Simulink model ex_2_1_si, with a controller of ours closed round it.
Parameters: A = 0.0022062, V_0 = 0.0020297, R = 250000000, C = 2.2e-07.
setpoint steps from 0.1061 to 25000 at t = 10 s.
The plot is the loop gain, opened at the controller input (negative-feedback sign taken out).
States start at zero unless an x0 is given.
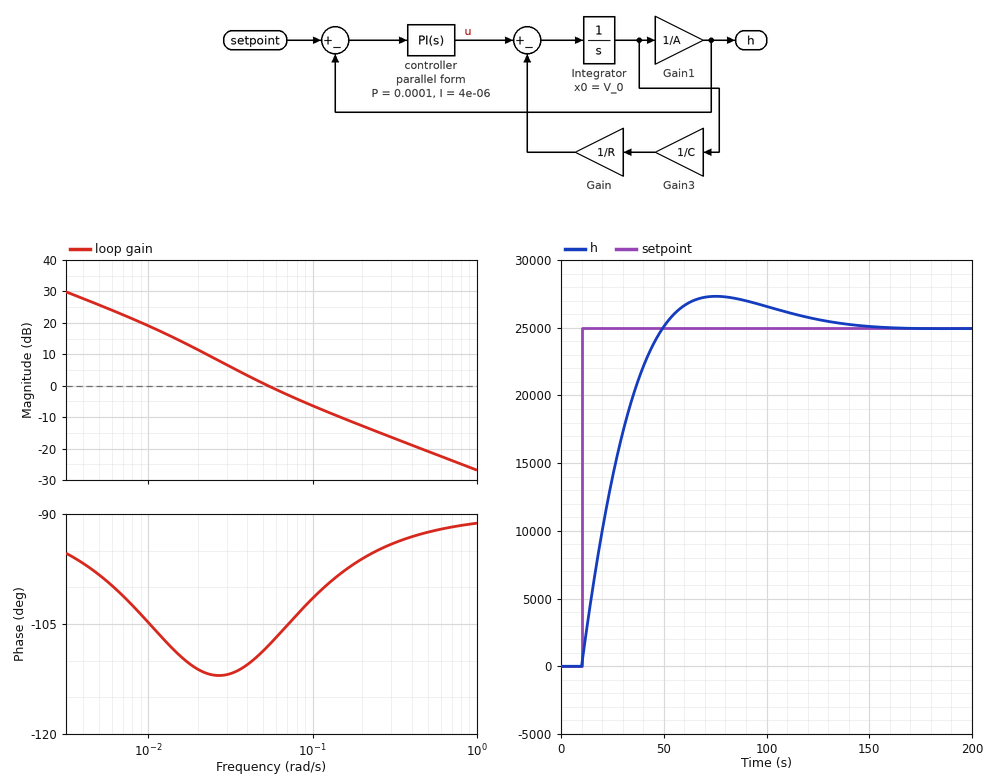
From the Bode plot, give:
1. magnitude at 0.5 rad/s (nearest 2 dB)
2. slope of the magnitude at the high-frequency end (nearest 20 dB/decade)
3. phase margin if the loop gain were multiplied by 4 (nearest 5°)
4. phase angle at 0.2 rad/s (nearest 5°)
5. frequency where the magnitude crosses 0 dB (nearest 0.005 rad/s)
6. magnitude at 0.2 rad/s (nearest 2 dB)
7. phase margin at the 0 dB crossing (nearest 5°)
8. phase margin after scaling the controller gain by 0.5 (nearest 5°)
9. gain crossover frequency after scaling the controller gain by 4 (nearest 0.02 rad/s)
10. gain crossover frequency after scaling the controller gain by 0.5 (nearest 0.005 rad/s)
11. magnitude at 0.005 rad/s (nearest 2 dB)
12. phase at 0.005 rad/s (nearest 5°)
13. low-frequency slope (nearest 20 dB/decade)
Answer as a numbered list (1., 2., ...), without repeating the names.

1. -20 dB
2. -20 dB/decade
3. 85°
4. -95°
5. 0.055 rad/s
6. -12 dB
7. 70°
8. 70°
9. 0.18 rad/s
10. 0.030 rad/s
11. 26 dB
12. -100°
13. -20 dB/decade
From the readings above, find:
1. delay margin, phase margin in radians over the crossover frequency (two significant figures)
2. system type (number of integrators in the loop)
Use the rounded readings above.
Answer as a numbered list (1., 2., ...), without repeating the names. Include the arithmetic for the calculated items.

1. 70 × π / 180 / 0.055 = 22 s
2. 1
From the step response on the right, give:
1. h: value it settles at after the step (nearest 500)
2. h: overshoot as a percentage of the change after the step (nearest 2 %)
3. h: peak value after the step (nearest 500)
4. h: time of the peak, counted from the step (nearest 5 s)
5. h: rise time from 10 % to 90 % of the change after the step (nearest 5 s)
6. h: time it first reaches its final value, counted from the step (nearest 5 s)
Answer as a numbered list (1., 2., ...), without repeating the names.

1. 25000
2. 10 %
3. 27500
4. 65 s
5. 30 s
6. 40 s
